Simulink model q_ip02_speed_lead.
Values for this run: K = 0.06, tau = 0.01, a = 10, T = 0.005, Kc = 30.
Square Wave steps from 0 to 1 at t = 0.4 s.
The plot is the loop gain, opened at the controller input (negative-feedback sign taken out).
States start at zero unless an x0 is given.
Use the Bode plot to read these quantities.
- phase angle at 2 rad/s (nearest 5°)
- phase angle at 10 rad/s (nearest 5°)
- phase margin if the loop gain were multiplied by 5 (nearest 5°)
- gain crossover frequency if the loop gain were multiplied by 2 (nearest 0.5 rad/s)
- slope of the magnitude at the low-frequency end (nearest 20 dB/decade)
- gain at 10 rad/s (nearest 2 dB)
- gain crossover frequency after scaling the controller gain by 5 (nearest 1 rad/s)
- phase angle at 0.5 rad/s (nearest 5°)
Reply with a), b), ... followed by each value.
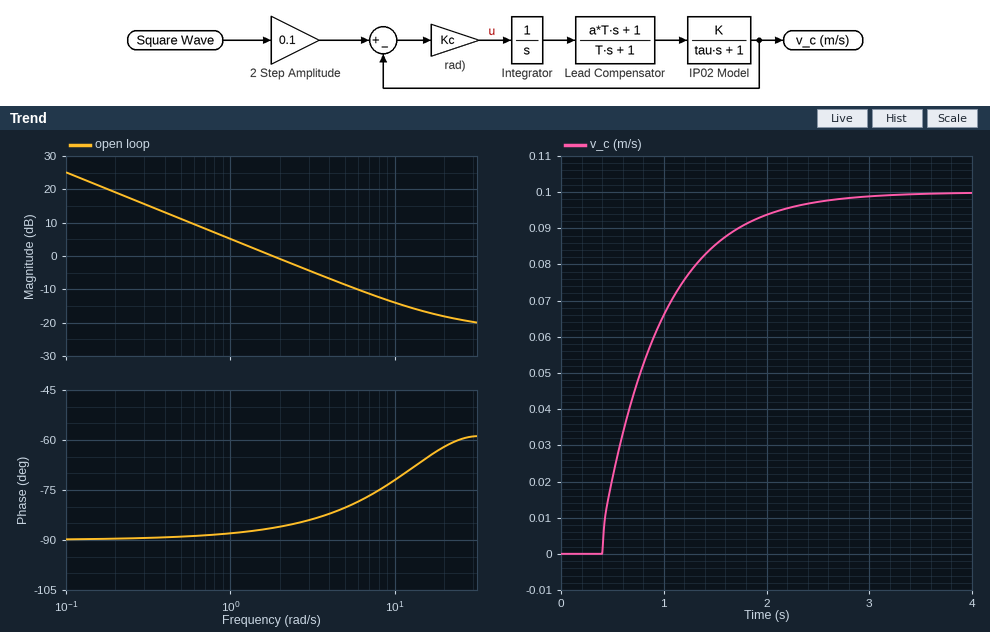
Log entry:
a) -85°
b) -70°
c) 110°
d) 3.5 rad/s
e) -20 dB/decade
f) -14 dB
g) 10 rad/s
h) -90°
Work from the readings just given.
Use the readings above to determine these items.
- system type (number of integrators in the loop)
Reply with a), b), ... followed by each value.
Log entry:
a) 1
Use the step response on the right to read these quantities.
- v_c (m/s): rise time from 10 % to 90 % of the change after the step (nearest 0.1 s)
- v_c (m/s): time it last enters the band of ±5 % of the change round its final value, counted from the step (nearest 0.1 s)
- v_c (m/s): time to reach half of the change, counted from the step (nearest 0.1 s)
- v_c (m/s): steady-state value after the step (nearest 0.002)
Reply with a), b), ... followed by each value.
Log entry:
a) 1.3 s
b) 1.7 s
c) 0.4 s
d) 0.100
